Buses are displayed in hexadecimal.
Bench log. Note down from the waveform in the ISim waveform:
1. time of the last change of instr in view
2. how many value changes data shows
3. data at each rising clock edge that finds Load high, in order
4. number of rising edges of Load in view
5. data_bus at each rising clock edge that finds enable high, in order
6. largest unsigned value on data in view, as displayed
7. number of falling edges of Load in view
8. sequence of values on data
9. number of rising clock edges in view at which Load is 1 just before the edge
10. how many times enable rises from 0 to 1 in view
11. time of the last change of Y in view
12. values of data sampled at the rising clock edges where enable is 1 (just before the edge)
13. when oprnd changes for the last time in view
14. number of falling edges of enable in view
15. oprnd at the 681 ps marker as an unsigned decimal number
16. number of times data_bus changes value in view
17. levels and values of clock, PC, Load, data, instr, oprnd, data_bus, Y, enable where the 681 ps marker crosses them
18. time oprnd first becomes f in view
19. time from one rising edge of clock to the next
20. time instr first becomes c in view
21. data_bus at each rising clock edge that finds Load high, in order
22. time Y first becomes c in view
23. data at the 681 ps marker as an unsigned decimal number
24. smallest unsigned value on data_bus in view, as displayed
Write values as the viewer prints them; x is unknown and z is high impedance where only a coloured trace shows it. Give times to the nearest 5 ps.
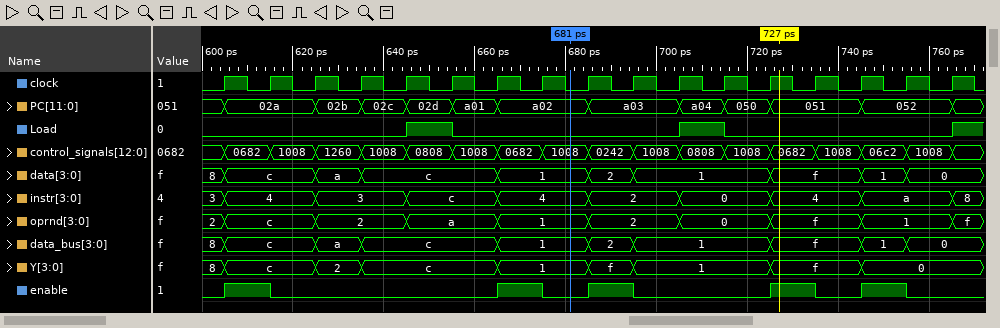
765 ps
9
c, 1
3
c, 1, 2, f, 1
f
2
8, c, a, c, 1, 2, 1, f, 1, 0
2
5
745 ps
c, 1, 2, f, 1
765 ps
5
1
9
clock=0, PC=a02, Load=0, data=1, instr=4, oprnd=1, data_bus=1, Y=1, enable=0
725 ps
10 ps
645 ps
c, 1
605 ps
1
0
